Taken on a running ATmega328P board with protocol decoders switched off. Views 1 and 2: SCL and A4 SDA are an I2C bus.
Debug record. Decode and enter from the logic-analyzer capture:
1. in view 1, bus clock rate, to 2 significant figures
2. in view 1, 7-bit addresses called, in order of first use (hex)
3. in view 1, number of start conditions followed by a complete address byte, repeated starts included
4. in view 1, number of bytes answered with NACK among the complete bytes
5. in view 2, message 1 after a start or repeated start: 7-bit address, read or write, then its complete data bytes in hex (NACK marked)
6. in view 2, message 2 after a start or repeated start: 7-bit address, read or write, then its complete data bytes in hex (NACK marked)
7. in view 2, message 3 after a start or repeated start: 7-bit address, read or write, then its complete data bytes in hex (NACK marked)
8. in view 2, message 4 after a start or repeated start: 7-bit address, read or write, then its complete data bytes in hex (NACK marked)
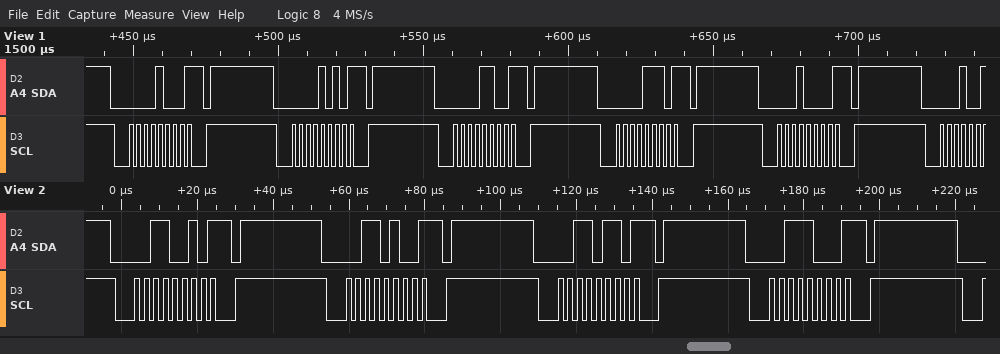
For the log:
400 kHz
0x04 0x05 0x06 0x07 0x08
5
5
0x19 write NACK
0x1A write NACK
0x1B write NACK
0x1C write NACK
